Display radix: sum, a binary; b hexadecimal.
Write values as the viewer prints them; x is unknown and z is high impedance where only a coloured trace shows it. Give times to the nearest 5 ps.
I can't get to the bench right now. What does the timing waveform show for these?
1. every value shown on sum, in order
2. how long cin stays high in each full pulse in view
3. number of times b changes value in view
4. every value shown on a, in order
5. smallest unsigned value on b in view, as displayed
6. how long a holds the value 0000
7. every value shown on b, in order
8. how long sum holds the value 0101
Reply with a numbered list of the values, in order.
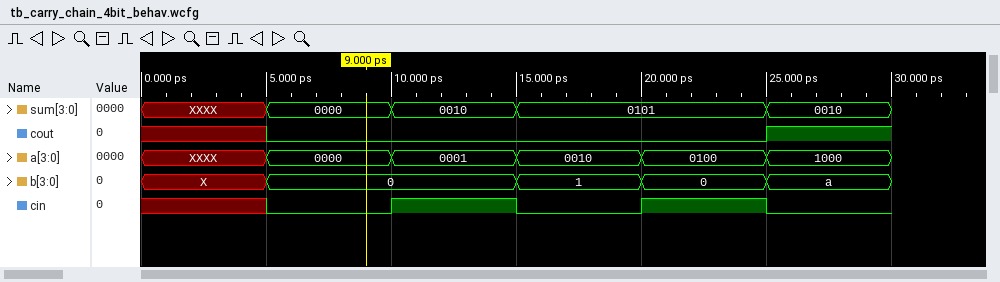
1. XXXX, 0000, 0010, 0101, 0010
2. 5 ps, 5 ps
3. 4
4. XXXX, 0000, 0001, 0010, 0100, 1000
5. 0
6. 5 ps
7. X, 0, 1, 0, a
8. 10 ps
